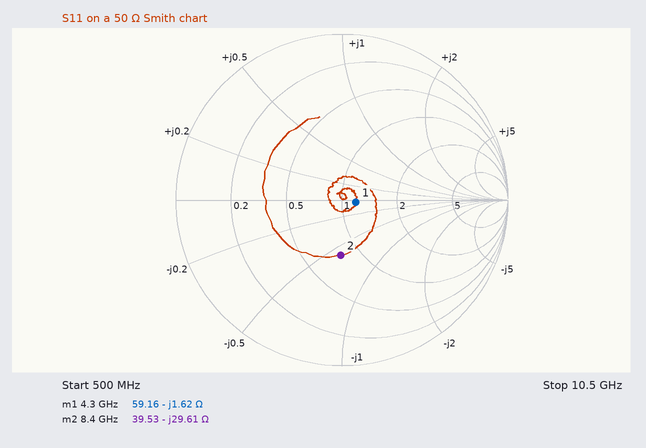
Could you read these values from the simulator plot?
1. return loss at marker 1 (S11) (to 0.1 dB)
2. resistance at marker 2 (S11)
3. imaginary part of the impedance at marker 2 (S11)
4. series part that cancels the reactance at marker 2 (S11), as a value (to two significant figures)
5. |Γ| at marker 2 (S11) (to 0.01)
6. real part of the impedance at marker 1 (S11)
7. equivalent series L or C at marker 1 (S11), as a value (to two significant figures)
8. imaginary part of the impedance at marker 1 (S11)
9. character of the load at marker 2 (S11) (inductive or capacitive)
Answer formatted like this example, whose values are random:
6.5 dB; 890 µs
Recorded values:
21.4 dB; 39.53 Ω; -29.61 Ω; 560 pH; 0.33; 59.16 Ω; 23 pF; -1.62 Ω; capacitive
